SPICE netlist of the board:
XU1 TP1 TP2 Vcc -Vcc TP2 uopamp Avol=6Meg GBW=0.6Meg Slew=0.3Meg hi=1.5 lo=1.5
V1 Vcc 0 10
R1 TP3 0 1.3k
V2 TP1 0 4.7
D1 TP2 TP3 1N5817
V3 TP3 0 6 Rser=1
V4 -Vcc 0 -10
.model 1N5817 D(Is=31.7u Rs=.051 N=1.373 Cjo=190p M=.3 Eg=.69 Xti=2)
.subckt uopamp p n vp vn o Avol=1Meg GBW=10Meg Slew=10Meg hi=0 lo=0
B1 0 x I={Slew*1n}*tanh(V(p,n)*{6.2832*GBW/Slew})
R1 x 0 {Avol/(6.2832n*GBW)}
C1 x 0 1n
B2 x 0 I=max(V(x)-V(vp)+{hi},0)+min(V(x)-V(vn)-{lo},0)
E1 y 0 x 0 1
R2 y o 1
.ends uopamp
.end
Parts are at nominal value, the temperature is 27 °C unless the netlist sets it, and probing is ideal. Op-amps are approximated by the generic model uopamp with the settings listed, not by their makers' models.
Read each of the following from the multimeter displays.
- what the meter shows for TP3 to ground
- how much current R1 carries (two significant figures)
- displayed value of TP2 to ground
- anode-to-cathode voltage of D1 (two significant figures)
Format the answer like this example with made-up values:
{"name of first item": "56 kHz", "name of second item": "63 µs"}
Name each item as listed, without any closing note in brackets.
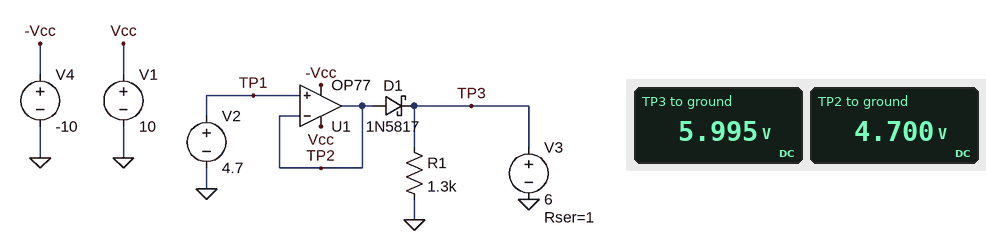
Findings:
{"what the meter shows for TP3 to ground": "5.995 V", "how much current R1 carries": "4.6 mA", "displayed value of TP2 to ground": "4.700 V", "anode-to-cathode voltage of D1": "-1.3 V"}
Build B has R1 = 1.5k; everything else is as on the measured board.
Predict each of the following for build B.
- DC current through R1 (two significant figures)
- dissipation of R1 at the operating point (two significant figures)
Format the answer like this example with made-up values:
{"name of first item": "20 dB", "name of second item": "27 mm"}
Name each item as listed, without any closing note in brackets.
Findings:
{"DC current through R1": "4.0 mA", "dissipation of R1 at the operating point": "24 mW"}
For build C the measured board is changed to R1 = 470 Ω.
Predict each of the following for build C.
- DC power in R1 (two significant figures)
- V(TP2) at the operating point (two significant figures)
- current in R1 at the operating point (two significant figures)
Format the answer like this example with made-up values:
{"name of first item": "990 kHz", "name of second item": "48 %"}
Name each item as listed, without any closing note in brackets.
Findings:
{"DC power in R1": "76 mW", "V(TP2) at the operating point": "4.7 V", "current in R1 at the operating point": "13 mA"}
